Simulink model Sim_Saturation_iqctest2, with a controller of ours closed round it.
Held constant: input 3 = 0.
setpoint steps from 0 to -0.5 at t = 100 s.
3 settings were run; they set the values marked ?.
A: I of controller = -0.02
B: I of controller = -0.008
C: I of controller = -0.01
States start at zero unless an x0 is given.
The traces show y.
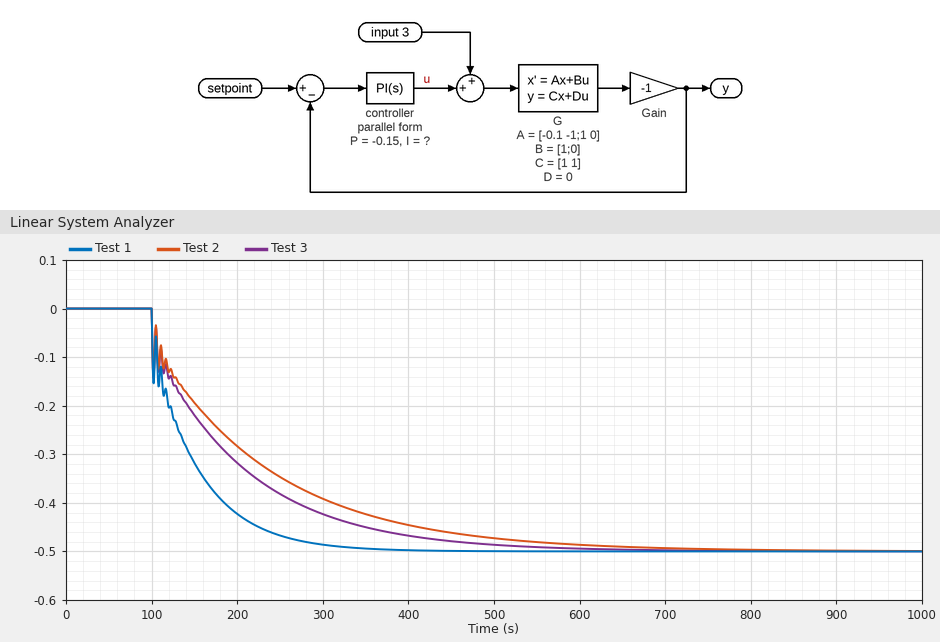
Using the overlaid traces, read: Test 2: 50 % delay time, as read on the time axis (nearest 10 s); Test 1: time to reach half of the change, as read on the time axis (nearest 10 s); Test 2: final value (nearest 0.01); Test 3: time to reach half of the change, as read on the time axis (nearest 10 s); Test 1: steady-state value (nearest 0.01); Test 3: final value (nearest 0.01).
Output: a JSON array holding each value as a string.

["180 s", "130 s", "-0.50", "160 s", "-0.50", "-0.50"]
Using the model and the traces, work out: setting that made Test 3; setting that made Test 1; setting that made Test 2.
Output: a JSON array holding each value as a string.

["C", "A", "B"]
